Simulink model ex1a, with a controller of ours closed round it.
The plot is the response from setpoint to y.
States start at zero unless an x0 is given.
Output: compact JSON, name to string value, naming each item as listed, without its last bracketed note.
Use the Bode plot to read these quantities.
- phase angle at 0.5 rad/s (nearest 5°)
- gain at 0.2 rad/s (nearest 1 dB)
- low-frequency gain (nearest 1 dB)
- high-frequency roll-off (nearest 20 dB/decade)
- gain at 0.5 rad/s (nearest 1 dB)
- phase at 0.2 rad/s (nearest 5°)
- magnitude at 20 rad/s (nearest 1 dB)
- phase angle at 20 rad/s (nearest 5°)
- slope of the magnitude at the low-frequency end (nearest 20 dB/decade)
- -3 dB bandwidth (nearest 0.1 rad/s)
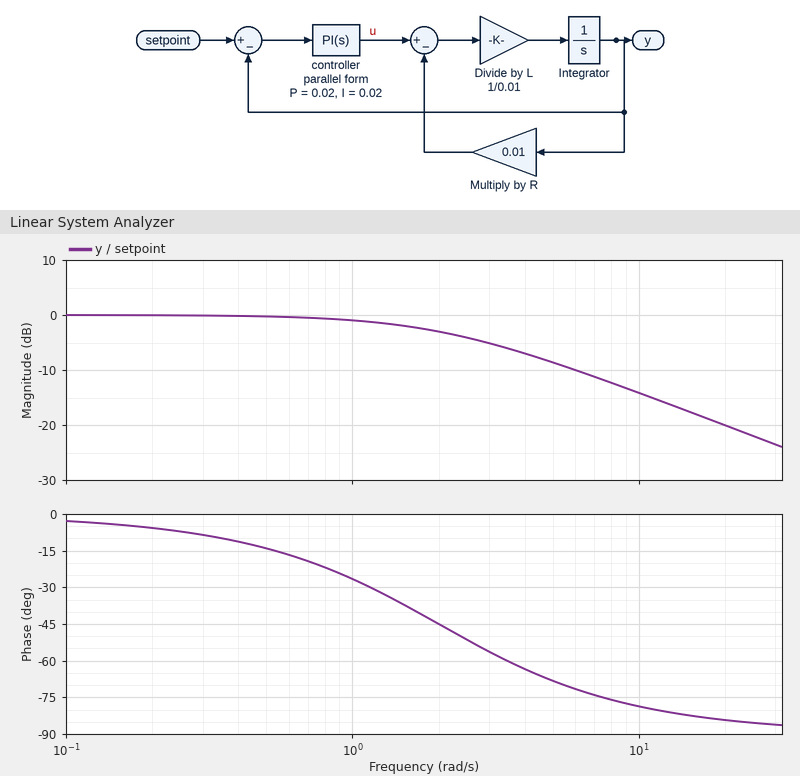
{"phase angle at 0.5 rad/s": "-15°", "gain at 0.2 rad/s": "0 dB", "low-frequency gain": "0 dB", "high-frequency roll-off": "-20 dB/decade", "gain at 0.5 rad/s": "0 dB", "phase at 0.2 rad/s": "-5°", "magnitude at 20 rad/s": "-20 dB", "phase angle at 20 rad/s": "-85°", "slope of the magnitude at the low-frequency end": "0 dB/decade", "-3 dB bandwidth": "2.0 rad/s"}
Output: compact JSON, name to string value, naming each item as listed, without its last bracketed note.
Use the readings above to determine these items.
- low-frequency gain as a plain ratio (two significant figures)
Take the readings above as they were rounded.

{"low-frequency gain as a plain ratio": "1.0"}
